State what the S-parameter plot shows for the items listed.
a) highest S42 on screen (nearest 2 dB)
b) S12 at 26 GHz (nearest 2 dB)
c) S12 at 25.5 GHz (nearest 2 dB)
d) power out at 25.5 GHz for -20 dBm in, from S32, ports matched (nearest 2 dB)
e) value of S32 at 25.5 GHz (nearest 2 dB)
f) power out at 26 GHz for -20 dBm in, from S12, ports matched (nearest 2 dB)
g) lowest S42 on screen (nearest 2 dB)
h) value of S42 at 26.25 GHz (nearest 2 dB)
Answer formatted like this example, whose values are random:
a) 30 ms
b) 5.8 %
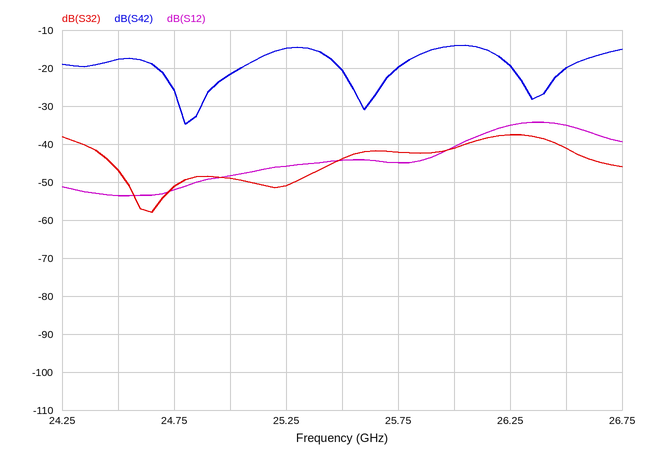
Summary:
a) -14 dB
b) -40 dB
c) -44 dB
d) -64 dBm
e) -44 dB
f) -60 dBm
g) -34 dB
h) -20 dB
